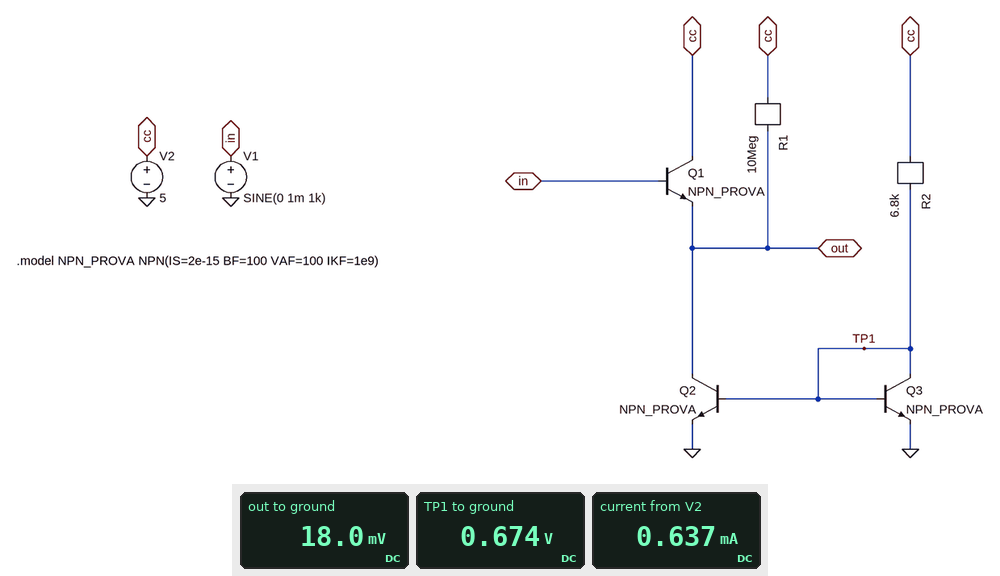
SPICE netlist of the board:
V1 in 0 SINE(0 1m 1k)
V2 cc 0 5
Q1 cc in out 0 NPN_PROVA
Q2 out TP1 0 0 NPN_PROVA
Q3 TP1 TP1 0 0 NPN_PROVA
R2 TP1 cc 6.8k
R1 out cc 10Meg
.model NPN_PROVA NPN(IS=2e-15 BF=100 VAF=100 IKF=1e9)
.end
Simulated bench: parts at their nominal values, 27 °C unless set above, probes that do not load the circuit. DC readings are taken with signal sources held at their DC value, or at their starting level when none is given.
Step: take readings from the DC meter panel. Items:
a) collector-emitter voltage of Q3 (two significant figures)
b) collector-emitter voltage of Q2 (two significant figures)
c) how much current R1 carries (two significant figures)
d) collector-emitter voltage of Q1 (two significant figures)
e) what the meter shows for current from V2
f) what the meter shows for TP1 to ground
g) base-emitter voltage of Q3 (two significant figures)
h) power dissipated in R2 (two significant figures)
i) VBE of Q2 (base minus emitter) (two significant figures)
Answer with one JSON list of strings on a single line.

["670 mV", "18 mV", "500 nA", "5.0 V", "0.637 mA", "0.674 V", "670 mV", "2.8 mW", "670 mV"]
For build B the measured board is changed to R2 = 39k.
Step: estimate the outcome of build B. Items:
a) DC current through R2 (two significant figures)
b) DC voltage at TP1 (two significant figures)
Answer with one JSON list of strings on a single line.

["110 µA", "630 mV"]
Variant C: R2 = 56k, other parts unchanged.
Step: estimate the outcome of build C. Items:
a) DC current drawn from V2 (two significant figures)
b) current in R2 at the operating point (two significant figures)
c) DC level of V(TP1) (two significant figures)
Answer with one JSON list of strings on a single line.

["79 µA", "78 µA", "620 mV"]
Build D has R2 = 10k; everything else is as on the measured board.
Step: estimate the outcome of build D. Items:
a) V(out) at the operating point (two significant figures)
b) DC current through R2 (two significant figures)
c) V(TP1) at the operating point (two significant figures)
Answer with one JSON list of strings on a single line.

["18 mV", "430 µA", "660 mV"]
